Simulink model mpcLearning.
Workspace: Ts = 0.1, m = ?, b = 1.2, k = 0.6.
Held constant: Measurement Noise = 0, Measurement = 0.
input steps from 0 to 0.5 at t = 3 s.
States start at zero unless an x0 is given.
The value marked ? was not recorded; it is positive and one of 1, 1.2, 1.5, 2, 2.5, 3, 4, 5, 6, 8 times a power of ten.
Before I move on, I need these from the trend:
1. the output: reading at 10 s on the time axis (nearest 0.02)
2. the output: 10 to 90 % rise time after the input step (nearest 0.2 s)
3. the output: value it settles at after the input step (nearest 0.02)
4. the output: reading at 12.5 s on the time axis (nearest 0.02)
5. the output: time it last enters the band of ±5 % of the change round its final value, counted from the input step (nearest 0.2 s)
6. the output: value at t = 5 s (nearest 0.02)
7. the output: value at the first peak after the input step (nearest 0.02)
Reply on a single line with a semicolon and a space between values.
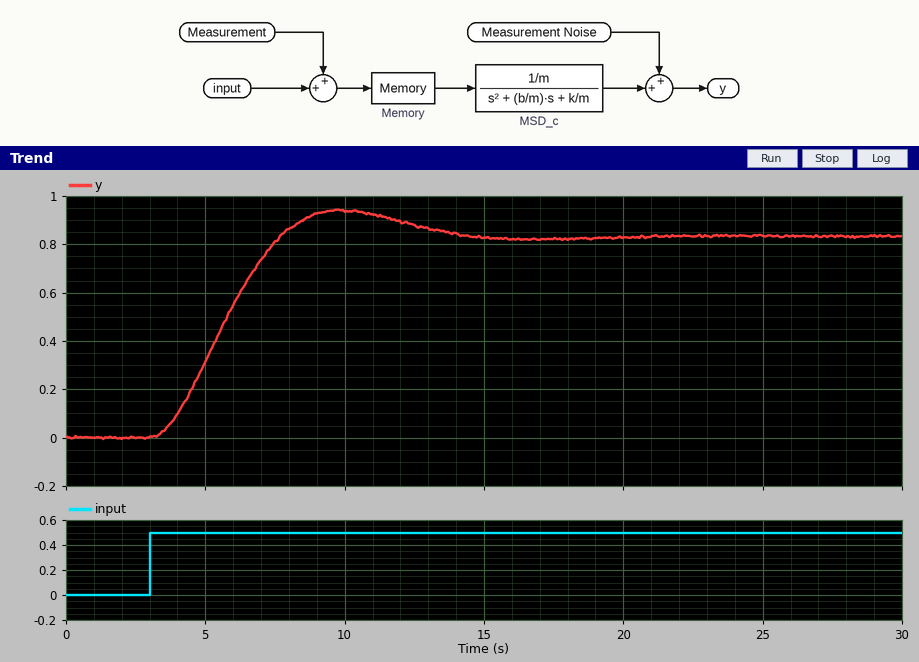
0.94; 3.2 s; 0.84; 0.88; 9.6 s; 0.32; 0.94
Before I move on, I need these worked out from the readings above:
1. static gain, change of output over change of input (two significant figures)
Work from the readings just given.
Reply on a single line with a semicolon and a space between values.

1.7
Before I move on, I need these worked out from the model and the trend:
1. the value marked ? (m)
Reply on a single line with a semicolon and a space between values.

2
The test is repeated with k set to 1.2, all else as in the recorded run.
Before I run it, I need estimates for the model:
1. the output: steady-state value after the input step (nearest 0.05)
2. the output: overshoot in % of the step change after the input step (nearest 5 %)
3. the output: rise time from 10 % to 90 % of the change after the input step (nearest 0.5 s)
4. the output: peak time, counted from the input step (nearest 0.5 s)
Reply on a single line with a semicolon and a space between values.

0.40; 25 %; 2.0 s; 4.5 s
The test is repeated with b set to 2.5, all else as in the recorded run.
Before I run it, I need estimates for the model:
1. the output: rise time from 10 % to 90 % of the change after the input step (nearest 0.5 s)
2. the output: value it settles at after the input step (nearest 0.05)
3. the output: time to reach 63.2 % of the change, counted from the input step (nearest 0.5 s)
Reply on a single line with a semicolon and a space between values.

7.5 s; 0.85; 4.5 s
